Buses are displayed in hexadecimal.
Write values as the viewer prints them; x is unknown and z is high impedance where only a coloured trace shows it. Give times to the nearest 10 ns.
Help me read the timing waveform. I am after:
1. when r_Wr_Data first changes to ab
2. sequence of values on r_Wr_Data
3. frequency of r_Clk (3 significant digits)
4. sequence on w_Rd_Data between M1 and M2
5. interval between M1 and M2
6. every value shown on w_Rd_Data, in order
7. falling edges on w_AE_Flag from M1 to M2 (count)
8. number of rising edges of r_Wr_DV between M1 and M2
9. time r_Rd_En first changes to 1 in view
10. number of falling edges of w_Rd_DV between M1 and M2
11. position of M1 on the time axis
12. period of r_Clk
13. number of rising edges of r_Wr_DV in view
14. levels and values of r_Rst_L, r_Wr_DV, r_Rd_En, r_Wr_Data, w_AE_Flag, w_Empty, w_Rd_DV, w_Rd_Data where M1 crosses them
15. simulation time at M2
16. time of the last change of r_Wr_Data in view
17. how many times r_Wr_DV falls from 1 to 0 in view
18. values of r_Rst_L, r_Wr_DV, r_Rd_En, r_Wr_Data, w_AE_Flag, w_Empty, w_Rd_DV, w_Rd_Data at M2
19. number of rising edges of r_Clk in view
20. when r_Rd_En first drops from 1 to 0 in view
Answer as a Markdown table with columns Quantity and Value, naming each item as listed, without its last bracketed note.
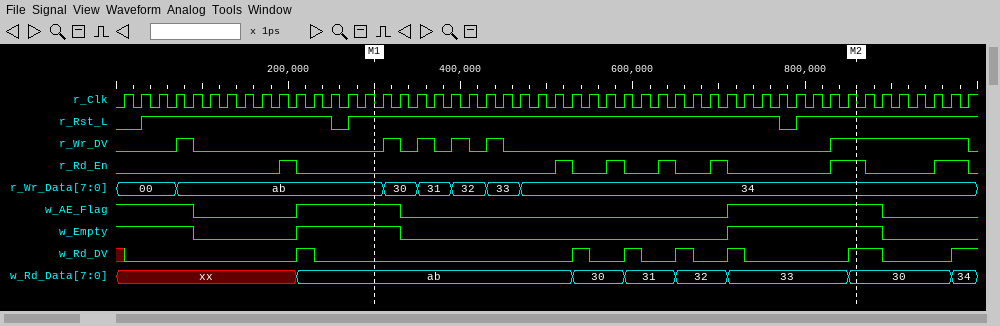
| Quantity | Value |
|---|---|
| when r_Wr_Data first changes to ab | 70 ns |
| sequence of values on r_Wr_Data | 00, ab, 30, 31, 32, 33, 34 |
| frequency of r_Clk | 50.0 MHz |
| sequence on w_Rd_Data between M1 and M2 | ab, 30, 31, 32, 33, 30 |
| interval between M1 and M2 | 560 ns |
| every value shown on w_Rd_Data, in order | xx, ab, 30, 31, 32, 33, 30, 34 |
| falling edges on w_AE_Flag from M1 to M2 | 1 |
| number of rising edges of r_Wr_DV between M1 and M2 | 5 |
| time r_Rd_En first changes to 1 in view | 190 ns |
| number of falling edges of w_Rd_DV between M1 and M2 | 4 |
| position of M1 on the time axis | 300 ns |
| period of r_Clk | 20 ns |
| number of rising edges of r_Wr_DV in view | 6 |
| levels and values of r_Rst_L, r_Wr_DV, r_Rd_En, r_Wr_Data, w_AE_Flag, w_Empty, w_Rd_DV, w_Rd_Data where M1 crosses them | r_Rst_L=1, r_Wr_DV=0, r_Rd_En=0, r_Wr_Data=ab, w_AE_Flag=1, w_Empty=1, w_Rd_DV=0, w_Rd_Data=ab |
| simulation time at M2 | 860 ns |
| time of the last change of r_Wr_Data in view | 470 ns |
| how many times r_Wr_DV falls from 1 to 0 in view | 6 |
| values of r_Rst_L, r_Wr_DV, r_Rd_En, r_Wr_Data, w_AE_Flag, w_Empty, w_Rd_DV, w_Rd_Data at M2 | r_Rst_L=1, r_Wr_DV=1, r_Rd_En=1, r_Wr_Data=34, w_AE_Flag=1, w_Empty=1, w_Rd_DV=1, w_Rd_Data=30 |
| number of rising edges of r_Clk in view | 50 |
| when r_Rd_En first drops from 1 to 0 in view | 210 ns |
